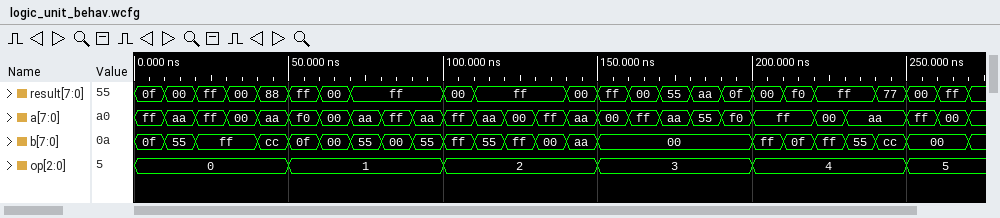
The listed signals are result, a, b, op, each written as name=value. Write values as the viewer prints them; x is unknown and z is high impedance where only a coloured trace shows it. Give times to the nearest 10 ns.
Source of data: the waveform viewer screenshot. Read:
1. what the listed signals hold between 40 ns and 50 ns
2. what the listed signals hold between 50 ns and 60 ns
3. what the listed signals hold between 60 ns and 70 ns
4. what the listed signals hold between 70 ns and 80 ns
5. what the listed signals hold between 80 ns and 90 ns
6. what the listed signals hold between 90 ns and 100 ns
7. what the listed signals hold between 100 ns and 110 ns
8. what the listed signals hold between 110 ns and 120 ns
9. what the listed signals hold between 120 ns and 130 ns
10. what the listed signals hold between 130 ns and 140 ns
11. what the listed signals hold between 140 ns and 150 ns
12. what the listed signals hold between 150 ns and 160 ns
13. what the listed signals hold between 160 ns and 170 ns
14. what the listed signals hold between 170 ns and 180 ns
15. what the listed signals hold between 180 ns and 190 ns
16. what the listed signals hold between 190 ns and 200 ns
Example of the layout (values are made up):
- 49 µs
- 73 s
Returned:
- result=88, a=aa, b=cc, op=0
- result=ff, a=f0, b=0f, op=1
- result=00, a=00, b=00, op=1
- result=ff, a=aa, b=55, op=1
- result=ff, a=ff, b=00, op=1
- result=ff, a=aa, b=55, op=1
- result=00, a=ff, b=ff, op=2
- result=ff, a=aa, b=55, op=2
- result=ff, a=00, b=ff, op=2
- result=ff, a=ff, b=00, op=2
- result=00, a=aa, b=aa, op=2
- result=ff, a=00, b=00, op=3
- result=00, a=ff, b=00, op=3
- result=55, a=aa, b=00, op=3
- result=aa, a=55, b=00, op=3
- result=0f, a=f0, b=00, op=3
